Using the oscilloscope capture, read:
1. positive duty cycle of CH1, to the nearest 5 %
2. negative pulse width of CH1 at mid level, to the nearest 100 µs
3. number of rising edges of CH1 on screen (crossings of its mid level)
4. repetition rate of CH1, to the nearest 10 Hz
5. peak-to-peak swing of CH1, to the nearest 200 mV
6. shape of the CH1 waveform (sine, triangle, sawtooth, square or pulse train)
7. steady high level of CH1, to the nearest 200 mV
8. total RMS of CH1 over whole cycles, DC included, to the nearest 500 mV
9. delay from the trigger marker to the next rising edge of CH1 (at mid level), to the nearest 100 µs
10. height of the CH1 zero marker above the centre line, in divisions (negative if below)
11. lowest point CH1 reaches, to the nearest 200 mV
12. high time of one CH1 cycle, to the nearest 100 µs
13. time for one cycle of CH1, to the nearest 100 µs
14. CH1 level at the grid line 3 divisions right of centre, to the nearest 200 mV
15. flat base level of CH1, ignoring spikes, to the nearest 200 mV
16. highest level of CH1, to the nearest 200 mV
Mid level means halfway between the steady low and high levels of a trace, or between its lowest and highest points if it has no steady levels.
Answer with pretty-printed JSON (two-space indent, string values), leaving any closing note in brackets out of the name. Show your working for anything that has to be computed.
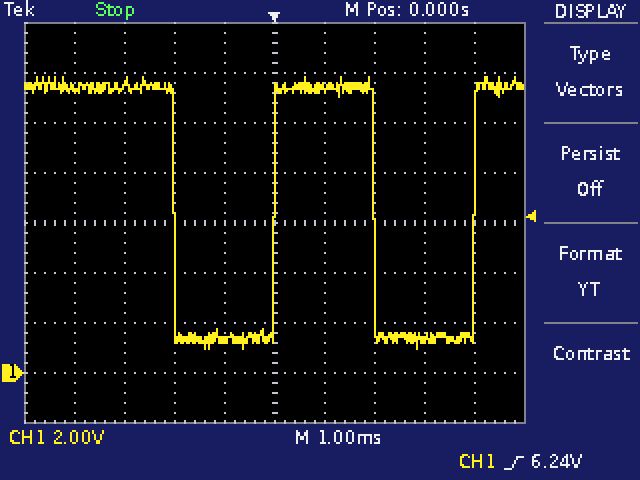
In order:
{
  "positive duty cycle of CH1, to the nearest 5 %": "2.0 ms / 4.0 ms ≈ 50 %",
  "negative pulse width of CH1 at mid level, to the nearest 100 µs": "2.0 ms",
  "number of rising edges of CH1 on screen": "2",
  "repetition rate of CH1, to the nearest 10 Hz": "1 / 4.0 ms ≈ 250 Hz",
  "peak-to-peak swing of CH1, to the nearest 200 mV": "11.8 V − (1.0 V) = 10.8 V",
  "shape of the CH1 waveform": "square",
  "steady high level of CH1, to the nearest 200 mV": "11.4 V",
  "total RMS of CH1 over whole cycles, DC included, to the nearest 500 mV": "√(0.5 × (11.4 V)² + 0.5 × (1.4 V)²) ≈ 8.12 V, so 8.0 V to the nearest 500 mV",
  "delay from the trigger marker to the next rising edge of CH1 (at mid level), to the nearest 100 µs": "4.0 ms",
  "height of the CH1 zero marker above the centre line, in divisions": "-3.0 div",
  "lowest point CH1 reaches, to the nearest 200 mV": "1.0 V",
  "high time of one CH1 cycle, to the nearest 100 µs": "2.0 ms",
  "time for one cycle of CH1, to the nearest 100 µs": "4.0 ms",
  "CH1 level at the grid line 3 divisions right of centre, to the nearest 200 mV": "1.4 V",
  "flat base level of CH1, ignoring spikes, to the nearest 200 mV": "1.4 V",
  "highest level of CH1, to the nearest 200 mV": "11.8 V"
}
